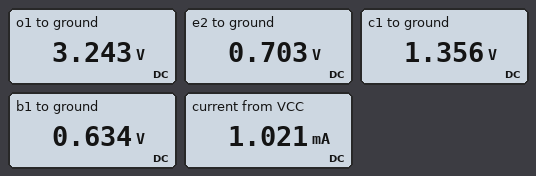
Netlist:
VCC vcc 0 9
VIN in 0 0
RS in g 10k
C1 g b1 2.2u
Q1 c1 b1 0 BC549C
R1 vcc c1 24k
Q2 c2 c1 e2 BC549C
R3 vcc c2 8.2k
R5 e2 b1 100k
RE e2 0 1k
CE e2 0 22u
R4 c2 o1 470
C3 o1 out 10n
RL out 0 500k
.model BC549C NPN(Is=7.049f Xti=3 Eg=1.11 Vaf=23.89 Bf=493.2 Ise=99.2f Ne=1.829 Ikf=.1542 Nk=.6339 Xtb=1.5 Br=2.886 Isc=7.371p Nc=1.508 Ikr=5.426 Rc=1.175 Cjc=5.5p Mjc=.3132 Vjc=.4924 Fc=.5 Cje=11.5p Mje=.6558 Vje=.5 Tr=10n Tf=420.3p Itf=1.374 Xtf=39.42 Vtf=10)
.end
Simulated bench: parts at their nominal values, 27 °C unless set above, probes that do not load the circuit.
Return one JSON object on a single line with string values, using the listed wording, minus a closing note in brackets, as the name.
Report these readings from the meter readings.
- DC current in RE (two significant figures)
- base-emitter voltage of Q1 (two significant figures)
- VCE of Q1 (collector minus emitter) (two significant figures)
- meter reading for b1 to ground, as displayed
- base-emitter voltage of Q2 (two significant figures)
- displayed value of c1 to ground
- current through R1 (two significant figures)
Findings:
{"DC current in RE": "700 µA", "base-emitter voltage of Q1": "630 mV", "VCE of Q1 (collector minus emitter)": "1.4 V", "meter reading for b1 to ground, as displayed": "0.634 V", "base-emitter voltage of Q2": "650 mV", "displayed value of c1 to ground": "1.356 V", "current through R1": "320 µA"}
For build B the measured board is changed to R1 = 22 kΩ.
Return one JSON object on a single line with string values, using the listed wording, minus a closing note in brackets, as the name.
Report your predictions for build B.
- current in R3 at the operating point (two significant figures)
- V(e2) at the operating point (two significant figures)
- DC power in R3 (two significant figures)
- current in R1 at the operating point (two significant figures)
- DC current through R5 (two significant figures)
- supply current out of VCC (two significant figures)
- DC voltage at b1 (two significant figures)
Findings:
{"current in R3 at the operating point": "710 µA", "V(e2) at the operating point": "710 mV", "DC power in R3": "4.1 mW", "current in R1 at the operating point": "350 µA", "DC current through R5": "750 nA", "supply current out of VCC": "1.1 mA", "DC voltage at b1": "640 mV"}
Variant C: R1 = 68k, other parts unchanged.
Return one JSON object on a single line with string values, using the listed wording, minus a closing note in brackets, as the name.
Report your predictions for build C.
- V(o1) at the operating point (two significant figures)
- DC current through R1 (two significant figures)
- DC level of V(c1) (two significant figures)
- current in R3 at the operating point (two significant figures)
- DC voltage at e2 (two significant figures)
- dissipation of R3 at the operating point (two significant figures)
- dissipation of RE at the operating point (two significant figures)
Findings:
{"V(o1) at the operating point": "3.8 V", "DC current through R1": "110 µA", "DC level of V(c1)": "1.3 V", "current in R3 at the operating point": "630 µA", "DC voltage at e2": "630 mV", "dissipation of R3 at the operating point": "3.3 mW", "dissipation of RE at the operating point": "400 µW"}
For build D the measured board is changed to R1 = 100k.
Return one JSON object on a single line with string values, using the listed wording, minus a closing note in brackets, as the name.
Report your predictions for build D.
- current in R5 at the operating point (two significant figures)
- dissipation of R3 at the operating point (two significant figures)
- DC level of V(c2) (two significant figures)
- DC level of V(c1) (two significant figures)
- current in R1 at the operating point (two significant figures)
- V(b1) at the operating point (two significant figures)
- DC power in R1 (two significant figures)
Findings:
{"current in R5 at the operating point": "180 nA", "dissipation of R3 at the operating point": "3.1 mW", "DC level of V(c2)": "4.0 V", "DC level of V(c1)": "1.3 V", "current in R1 at the operating point": "77 µA", "V(b1) at the operating point": "600 mV", "DC power in R1": "600 µW"}
